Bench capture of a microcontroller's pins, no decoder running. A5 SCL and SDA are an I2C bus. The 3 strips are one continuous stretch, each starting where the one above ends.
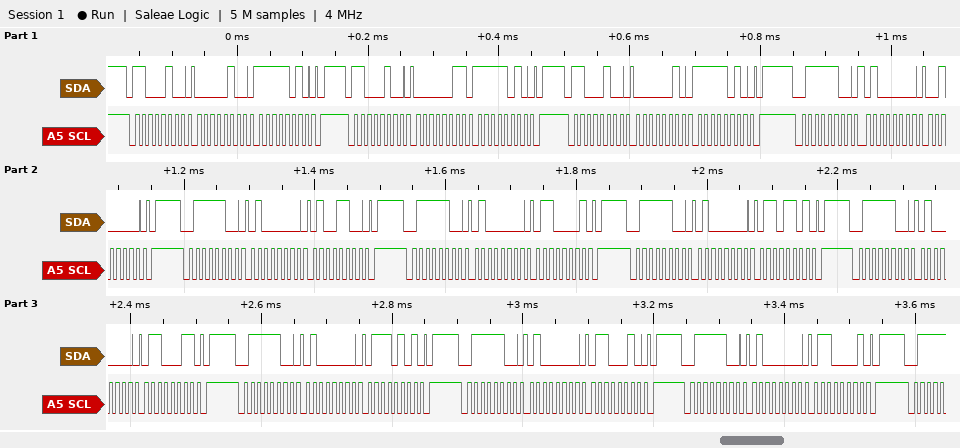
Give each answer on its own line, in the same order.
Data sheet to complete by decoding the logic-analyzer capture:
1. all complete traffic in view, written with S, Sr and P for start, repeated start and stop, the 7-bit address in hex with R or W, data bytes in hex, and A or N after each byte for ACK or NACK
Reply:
S 62W A 04 A FA A P S 62W A 03 A FA A P S 62W A 02 A FA A P S 3EW A 40 A 20 A P S 3EW A 40 A 4C A P S 3EW A 40 A 61 A P S 3EW A 40 A 6D A P S 3EW A 40 A 63 A P S 3EW A 40 A 75 A P S 3EW A 40 A 62 A P S 3EW A 40 A 61 A P
